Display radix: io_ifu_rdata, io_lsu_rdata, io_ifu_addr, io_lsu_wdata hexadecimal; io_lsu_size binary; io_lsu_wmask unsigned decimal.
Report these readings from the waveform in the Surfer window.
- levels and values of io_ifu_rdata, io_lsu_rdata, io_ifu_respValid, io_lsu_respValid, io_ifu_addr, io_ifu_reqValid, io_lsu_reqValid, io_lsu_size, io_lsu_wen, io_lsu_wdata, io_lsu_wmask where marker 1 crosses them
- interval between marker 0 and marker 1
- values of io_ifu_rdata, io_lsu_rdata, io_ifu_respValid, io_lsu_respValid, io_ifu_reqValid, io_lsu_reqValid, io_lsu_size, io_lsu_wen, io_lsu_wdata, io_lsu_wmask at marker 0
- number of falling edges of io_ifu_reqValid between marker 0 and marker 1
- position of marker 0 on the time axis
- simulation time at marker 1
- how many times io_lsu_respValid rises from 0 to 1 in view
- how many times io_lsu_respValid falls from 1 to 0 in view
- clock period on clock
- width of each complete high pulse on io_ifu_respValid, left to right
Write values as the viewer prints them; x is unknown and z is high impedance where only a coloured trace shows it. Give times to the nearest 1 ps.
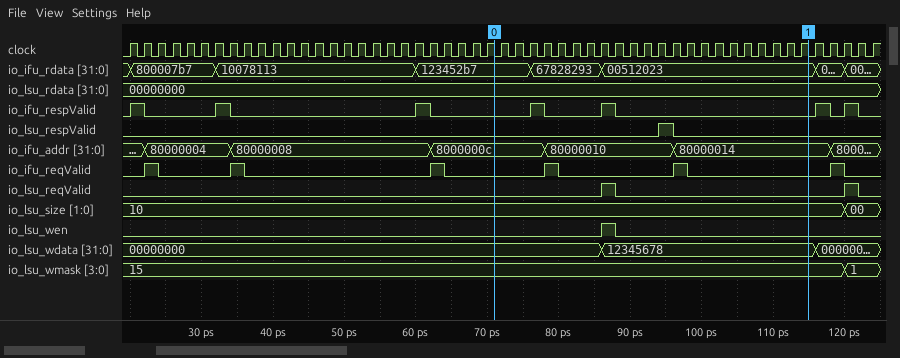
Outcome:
io_ifu_rdata=00512023, io_lsu_rdata=00000000, io_ifu_respValid=0, io_lsu_respValid=0, io_ifu_addr=80000014, io_ifu_reqValid=0, io_lsu_reqValid=0, io_lsu_size=10, io_lsu_wen=0, io_lsu_wdata=12345678, io_lsu_wmask=15
44 ps
io_ifu_rdata=123452b7, io_lsu_rdata=00000000, io_ifu_respValid=0, io_lsu_respValid=0, io_ifu_reqValid=0, io_lsu_reqValid=0, io_lsu_size=10, io_lsu_wen=0, io_lsu_wdata=00000000, io_lsu_wmask=15
2
71 ps
115 ps
1
1
2 ps
2 ps, 2 ps, 2 ps, 2 ps, 2 ps, 2 ps, 2 ps
